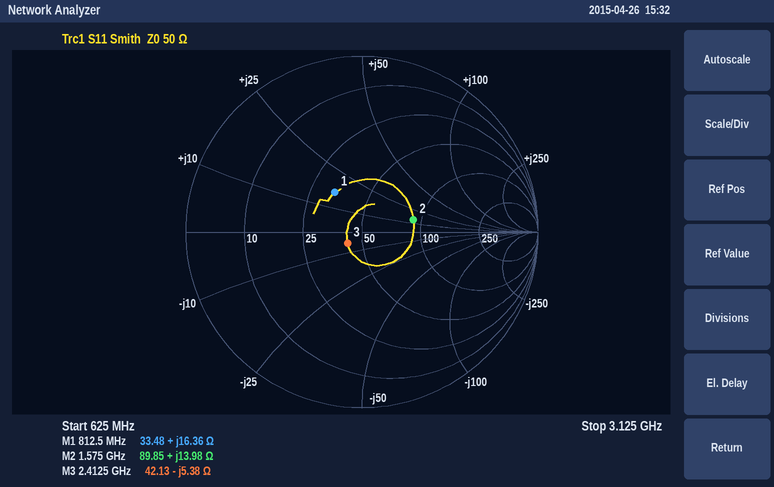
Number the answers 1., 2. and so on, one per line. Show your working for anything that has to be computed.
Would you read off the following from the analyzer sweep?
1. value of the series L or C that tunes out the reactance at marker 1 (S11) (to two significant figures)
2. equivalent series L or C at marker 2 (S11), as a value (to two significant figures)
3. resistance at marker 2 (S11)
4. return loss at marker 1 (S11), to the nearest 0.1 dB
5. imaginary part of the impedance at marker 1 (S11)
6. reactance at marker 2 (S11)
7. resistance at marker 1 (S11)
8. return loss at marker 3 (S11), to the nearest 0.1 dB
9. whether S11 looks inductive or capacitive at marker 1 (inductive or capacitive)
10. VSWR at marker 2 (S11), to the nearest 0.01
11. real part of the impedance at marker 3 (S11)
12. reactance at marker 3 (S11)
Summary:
1. C = 1/(2π × 812.5 MHz × 16.36 Ω) ≈ 12 pF
2. L = 13.98 Ω/(2π × 1.575 GHz) ≈ 1.4 nH
3. 89.85 Ω
4. 11.3 dB
5. +16.36 Ω
6. +13.98 Ω
7. 33.48 Ω
8. 19.7 dB
9. inductive
10. 1.86
11. 42.13 Ω
12. -5.38 Ω
